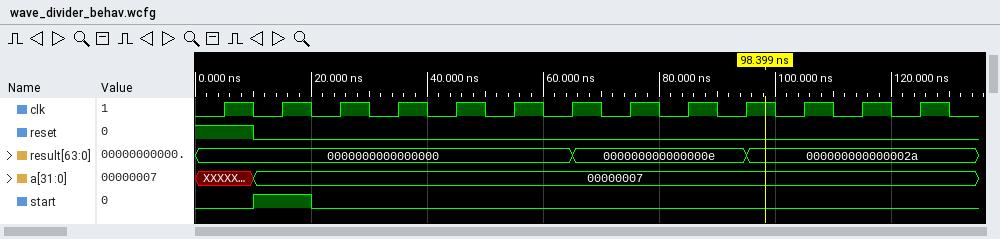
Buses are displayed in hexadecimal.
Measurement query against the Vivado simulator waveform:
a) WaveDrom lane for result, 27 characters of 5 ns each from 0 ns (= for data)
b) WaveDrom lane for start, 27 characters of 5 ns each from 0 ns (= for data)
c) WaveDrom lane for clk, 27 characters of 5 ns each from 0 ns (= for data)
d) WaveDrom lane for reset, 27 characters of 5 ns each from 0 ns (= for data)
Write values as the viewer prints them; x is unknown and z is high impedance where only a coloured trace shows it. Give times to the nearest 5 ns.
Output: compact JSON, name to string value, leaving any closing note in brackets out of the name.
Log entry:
{"WaveDrom lane for result, 27 characters of 5 ns each from 0 ns": "{name: 'result', wave: '=............=.....=.......', data: '0000000000000000 000000000000000e 000000000000002a'}", "WaveDrom lane for start, 27 characters of 5 ns each from 0 ns": "{name: 'start', wave: '0.1.0......................'}", "WaveDrom lane for clk, 27 characters of 5 ns each from 0 ns": "{name: 'clk', wave: '010101010101010101010101010'}", "WaveDrom lane for reset, 27 characters of 5 ns each from 0 ns": "{name: 'reset', wave: '1.0........................'}"}
